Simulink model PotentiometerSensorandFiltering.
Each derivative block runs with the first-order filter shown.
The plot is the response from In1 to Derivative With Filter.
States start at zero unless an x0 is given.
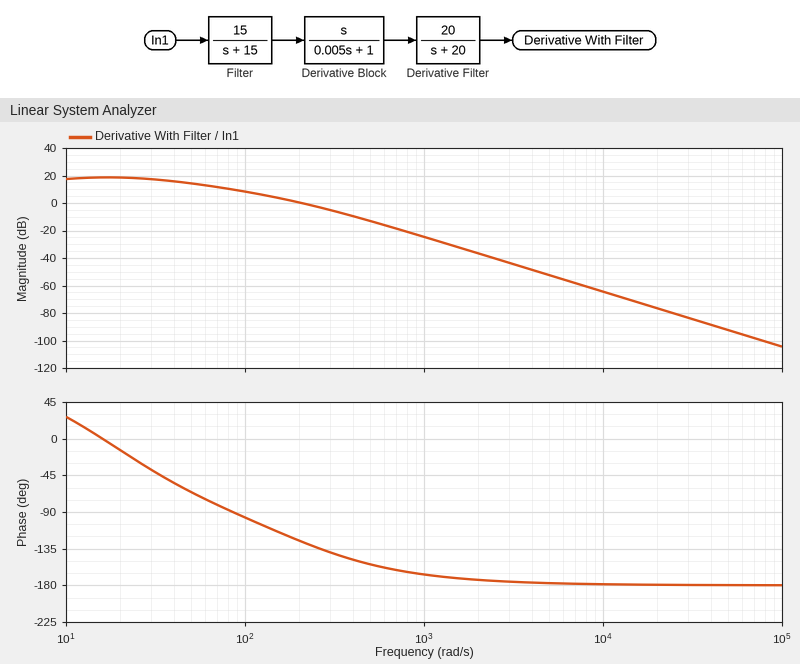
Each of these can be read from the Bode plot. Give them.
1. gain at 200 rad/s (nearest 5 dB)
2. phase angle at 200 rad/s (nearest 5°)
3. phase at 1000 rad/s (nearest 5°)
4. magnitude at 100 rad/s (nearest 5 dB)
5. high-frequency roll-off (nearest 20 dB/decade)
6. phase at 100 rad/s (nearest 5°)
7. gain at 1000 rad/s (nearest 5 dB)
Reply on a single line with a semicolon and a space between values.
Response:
0 dB; -125°; -165°; 10 dB; -40 dB/decade; -95°; -25 dB
